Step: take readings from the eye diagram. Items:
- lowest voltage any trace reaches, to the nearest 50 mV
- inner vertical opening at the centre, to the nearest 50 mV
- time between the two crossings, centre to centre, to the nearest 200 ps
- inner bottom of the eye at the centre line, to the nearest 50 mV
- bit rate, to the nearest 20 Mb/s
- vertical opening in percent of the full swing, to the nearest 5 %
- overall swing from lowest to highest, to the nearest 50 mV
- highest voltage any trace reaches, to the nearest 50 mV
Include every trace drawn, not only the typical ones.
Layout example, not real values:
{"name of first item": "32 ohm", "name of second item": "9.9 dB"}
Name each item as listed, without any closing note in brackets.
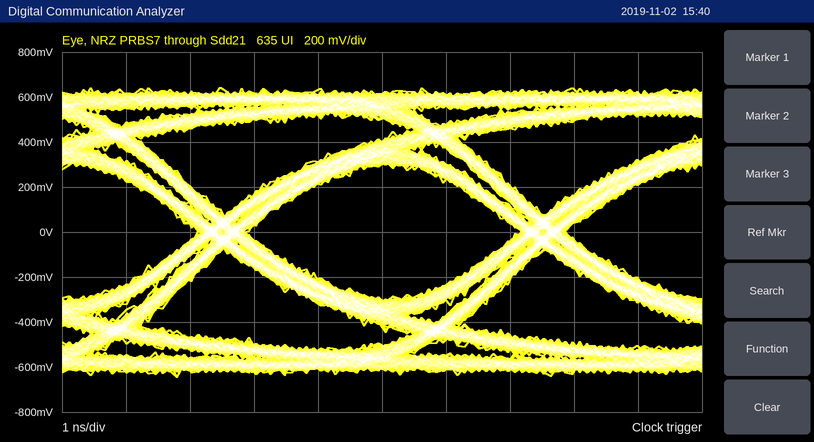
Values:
{"lowest voltage any trace reaches, to the nearest 50 mV": "-650 mV", "inner vertical opening at the centre, to the nearest 50 mV": "600 mV", "time between the two crossings, centre to centre, to the nearest 200 ps": "5.0 ns", "inner bottom of the eye at the centre line, to the nearest 50 mV": "-300 mV", "bit rate, to the nearest 20 Mb/s": "200 Mb/s", "vertical opening in percent of the full swing, to the nearest 5 %": "45 %", "overall swing from lowest to highest, to the nearest 50 mV": "1.30 V", "highest voltage any trace reaches, to the nearest 50 mV": "650 mV"}
